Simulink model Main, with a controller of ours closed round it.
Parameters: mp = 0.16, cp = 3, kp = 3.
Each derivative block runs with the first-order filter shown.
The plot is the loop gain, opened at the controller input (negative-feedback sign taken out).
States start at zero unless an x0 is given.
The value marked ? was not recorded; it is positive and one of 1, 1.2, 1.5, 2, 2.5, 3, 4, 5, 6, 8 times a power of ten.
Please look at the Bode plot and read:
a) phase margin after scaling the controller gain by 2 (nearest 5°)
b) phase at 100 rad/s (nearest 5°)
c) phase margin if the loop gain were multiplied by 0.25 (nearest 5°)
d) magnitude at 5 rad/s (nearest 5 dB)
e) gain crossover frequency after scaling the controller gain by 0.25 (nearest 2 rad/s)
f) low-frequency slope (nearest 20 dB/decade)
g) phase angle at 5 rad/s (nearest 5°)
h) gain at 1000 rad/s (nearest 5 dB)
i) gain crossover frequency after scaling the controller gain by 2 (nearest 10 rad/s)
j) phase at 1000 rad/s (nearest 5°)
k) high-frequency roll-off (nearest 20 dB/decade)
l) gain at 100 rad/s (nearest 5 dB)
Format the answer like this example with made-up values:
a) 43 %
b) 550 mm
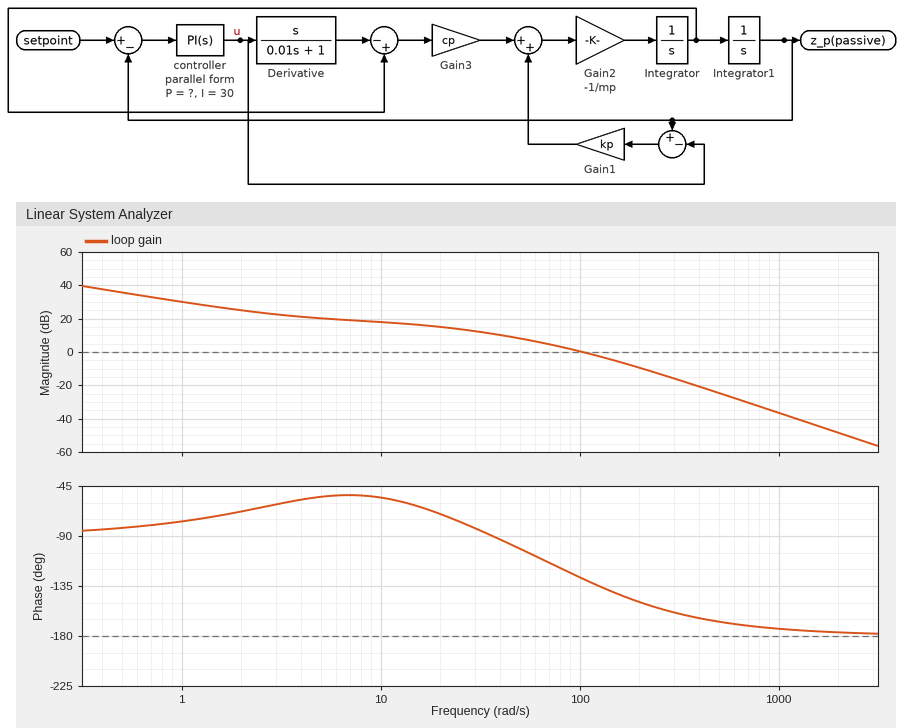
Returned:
a) 35°
b) -125°
c) 95°
d) 20 dB
e) 32 rad/s
f) -20 dB/decade
g) -55°
h) -35 dB
i) 160 rad/s
j) -175°
k) -40 dB/decade
l) 0 dB
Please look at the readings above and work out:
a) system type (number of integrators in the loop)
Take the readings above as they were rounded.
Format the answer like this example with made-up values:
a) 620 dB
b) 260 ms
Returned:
a) 1
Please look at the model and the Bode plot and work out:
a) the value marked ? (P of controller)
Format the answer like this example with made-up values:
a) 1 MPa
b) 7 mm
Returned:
a) 8
